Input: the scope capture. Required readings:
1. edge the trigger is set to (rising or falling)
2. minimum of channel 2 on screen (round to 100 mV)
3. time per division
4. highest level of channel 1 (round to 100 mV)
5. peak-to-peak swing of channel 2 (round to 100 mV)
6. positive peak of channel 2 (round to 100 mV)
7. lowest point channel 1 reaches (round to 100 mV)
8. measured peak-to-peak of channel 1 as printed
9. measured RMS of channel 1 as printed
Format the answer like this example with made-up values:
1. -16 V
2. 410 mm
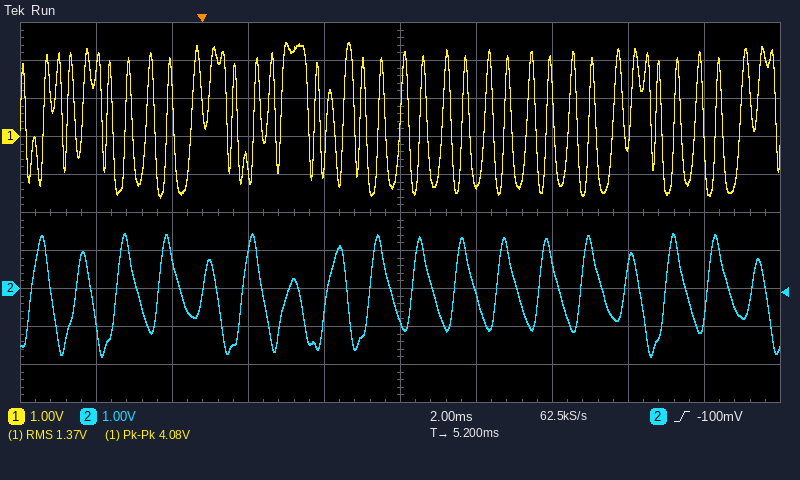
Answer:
1. rising
2. -1.8 V
3. 2 ms
4. 2.5 V
5. 3.2 V
6. 1.4 V
7. -1.6 V
8. 4.08 V
9. 1.37 V
